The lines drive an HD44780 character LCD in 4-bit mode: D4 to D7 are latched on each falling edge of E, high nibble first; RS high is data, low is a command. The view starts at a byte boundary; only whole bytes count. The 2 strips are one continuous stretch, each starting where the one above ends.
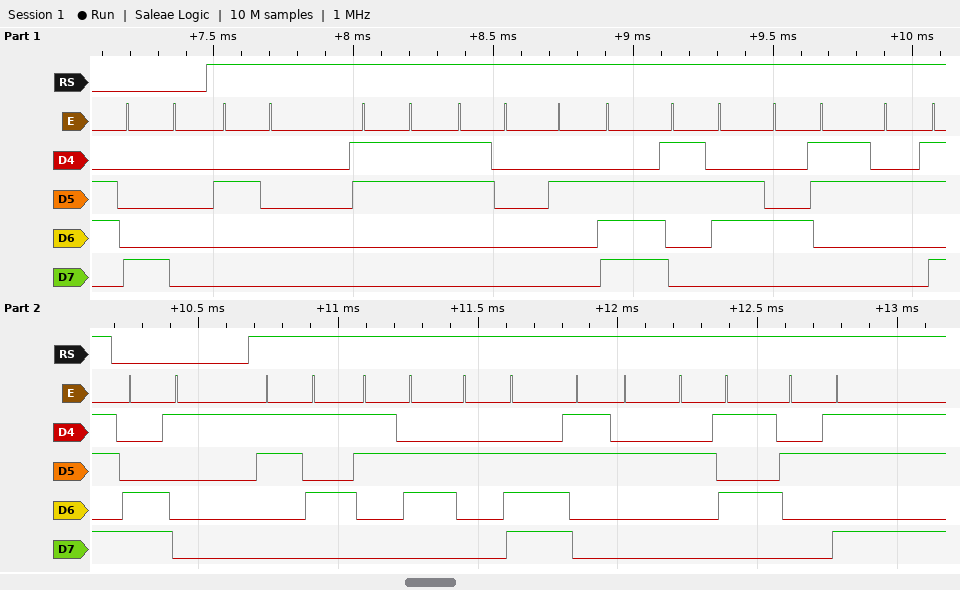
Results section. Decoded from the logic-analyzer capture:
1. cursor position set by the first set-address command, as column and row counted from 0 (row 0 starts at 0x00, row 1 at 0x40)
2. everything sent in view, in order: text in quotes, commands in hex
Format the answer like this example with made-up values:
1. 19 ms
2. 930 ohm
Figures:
1. column 0, row 0
2. 0x80 " 30.6C+" 0xC1 "56.2%+"
